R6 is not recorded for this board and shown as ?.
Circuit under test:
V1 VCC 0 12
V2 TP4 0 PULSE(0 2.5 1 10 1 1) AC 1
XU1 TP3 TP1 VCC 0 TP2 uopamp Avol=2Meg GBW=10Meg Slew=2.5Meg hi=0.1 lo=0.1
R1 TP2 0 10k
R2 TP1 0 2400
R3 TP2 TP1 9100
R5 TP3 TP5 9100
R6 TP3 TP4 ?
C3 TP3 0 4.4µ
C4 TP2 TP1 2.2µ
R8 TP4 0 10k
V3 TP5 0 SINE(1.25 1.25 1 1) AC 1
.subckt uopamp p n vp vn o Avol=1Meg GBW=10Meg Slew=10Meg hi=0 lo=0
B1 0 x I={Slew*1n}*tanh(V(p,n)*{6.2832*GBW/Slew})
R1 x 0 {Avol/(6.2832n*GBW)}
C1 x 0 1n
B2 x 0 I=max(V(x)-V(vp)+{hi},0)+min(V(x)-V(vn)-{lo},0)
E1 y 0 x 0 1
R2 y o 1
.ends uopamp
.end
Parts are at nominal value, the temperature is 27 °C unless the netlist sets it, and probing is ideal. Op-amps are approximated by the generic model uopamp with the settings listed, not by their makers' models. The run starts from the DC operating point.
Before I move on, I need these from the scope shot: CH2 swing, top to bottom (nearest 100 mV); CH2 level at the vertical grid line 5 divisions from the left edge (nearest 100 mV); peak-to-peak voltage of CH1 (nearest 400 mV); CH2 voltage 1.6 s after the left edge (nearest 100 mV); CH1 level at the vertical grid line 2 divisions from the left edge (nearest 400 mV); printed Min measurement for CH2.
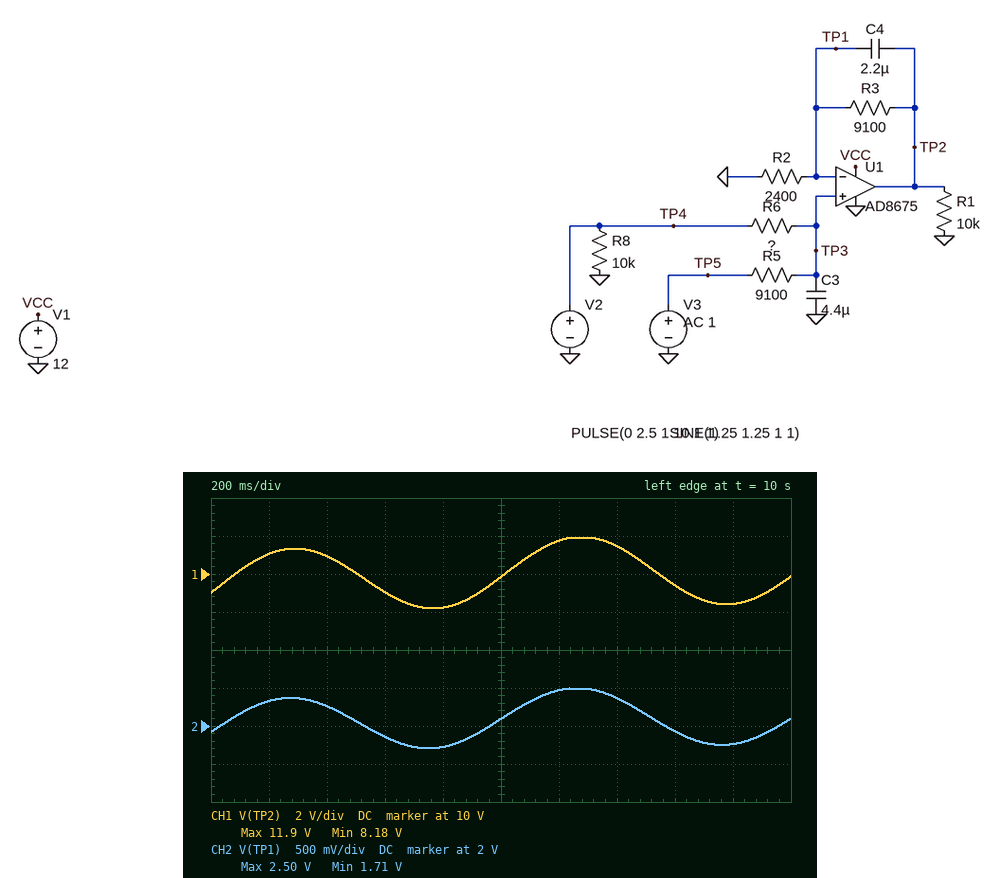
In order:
800 mV
2.1 V
3.6 V
1.9 V
10.8 V
1.71 V
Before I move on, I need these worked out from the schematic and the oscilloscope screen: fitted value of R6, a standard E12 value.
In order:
3.9 kΩ
